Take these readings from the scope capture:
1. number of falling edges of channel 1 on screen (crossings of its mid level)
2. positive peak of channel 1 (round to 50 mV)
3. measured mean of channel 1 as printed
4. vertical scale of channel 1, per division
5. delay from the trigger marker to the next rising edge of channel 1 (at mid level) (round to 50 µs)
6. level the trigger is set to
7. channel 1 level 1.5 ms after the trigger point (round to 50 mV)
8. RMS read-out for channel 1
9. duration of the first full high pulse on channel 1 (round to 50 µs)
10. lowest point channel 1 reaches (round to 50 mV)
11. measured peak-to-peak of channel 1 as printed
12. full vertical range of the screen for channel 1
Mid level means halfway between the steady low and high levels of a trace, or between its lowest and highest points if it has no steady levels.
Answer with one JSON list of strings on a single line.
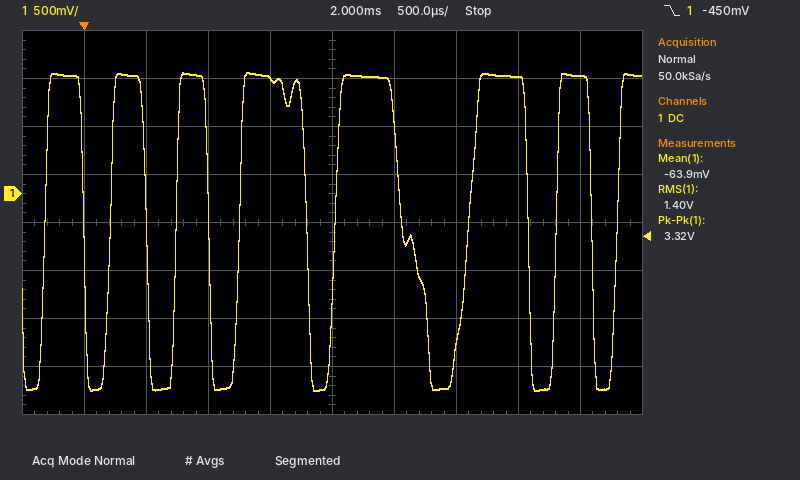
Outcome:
["7", "1.25 V", "-63.9 mV", "500 mV", "200 µs", "-450 mV", "1.20 V", "1.40 V", "300 µs", "-2.05 V", "3.32 V", "4 V"]
